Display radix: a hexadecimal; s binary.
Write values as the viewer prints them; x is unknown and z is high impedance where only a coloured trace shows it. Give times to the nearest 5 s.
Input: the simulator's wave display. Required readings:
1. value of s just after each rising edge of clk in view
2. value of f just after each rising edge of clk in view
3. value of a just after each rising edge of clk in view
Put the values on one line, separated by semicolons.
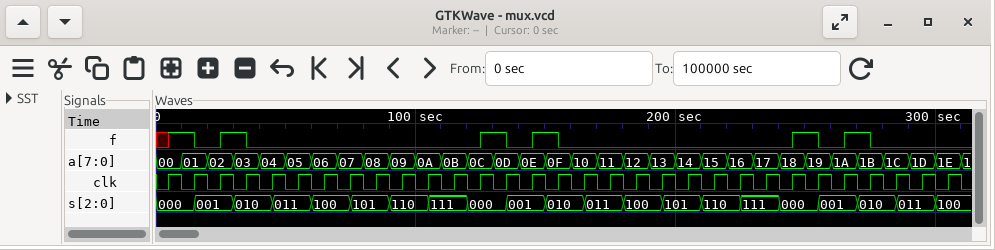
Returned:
000, 001, 001, 010, 011, 011, 100, 101, 101, 110, 111, 111, 000, 001, 001, 010, 011, 011, 100, 101, 101, 110, 111, 111, 000, 001, 001, 010, 011, 011, 100; 1 0 1 0 0 0 0 0 0 0 0 0 1 0 1 0 0 0 0 0 0 0 0 0 1 0 1 0 0 0 0; 00, 01, 02, 03, 04, 05, 06, 07, 08, 09, 0A, 0B, 0C, 0D, 0E, 0F, 10, 11, 12, 13, 14, 15, 16, 17, 18, 19, 1A, 1B, 1C, 1D, 1E
